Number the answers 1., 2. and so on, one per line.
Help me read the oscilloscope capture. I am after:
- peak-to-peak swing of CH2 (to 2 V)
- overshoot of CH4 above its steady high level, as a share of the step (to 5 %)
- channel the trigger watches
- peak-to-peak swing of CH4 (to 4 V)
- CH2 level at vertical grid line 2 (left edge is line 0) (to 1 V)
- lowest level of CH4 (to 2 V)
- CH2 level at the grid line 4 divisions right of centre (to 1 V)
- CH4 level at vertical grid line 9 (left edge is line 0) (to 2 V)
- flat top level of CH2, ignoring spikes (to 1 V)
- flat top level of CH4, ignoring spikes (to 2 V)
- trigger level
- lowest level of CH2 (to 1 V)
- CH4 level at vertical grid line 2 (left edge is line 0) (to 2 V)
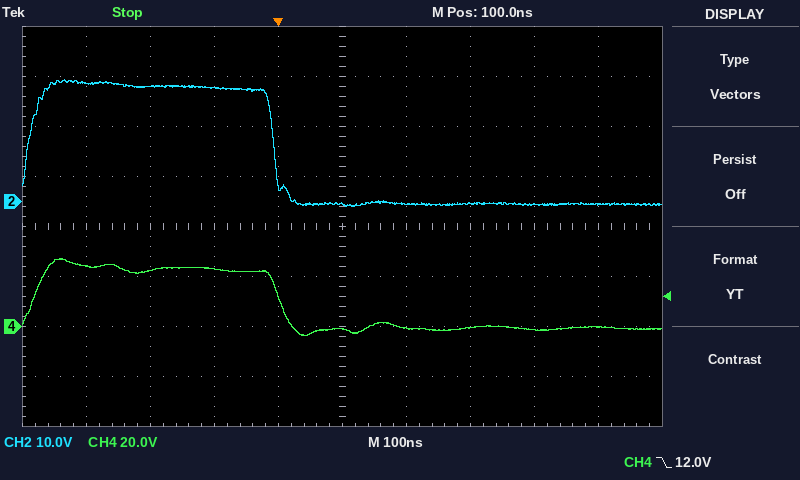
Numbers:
1. 26 V
2. 15 %
3. CH4
4. 32 V
5. 23 V
6. -4 V
7. -1 V
8. 0 V
9. 23 V
10. 24 V
11. 12.0 V
12. -1 V
13. 22 V
